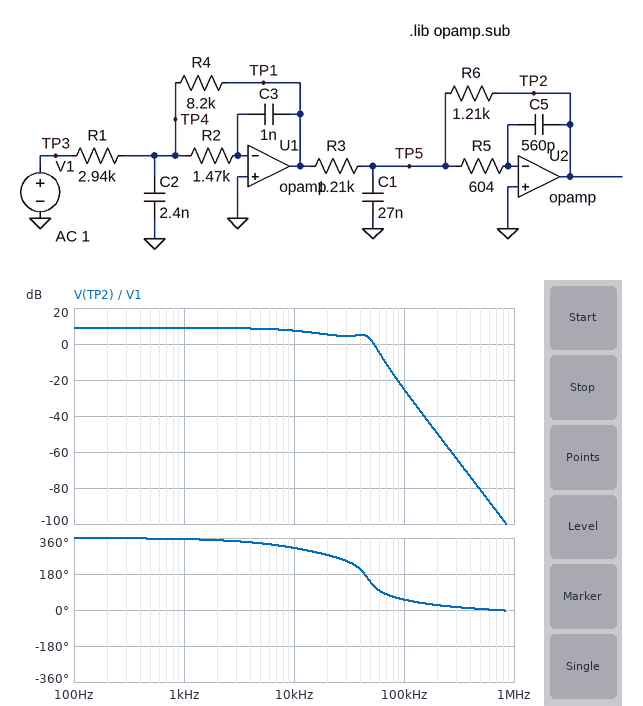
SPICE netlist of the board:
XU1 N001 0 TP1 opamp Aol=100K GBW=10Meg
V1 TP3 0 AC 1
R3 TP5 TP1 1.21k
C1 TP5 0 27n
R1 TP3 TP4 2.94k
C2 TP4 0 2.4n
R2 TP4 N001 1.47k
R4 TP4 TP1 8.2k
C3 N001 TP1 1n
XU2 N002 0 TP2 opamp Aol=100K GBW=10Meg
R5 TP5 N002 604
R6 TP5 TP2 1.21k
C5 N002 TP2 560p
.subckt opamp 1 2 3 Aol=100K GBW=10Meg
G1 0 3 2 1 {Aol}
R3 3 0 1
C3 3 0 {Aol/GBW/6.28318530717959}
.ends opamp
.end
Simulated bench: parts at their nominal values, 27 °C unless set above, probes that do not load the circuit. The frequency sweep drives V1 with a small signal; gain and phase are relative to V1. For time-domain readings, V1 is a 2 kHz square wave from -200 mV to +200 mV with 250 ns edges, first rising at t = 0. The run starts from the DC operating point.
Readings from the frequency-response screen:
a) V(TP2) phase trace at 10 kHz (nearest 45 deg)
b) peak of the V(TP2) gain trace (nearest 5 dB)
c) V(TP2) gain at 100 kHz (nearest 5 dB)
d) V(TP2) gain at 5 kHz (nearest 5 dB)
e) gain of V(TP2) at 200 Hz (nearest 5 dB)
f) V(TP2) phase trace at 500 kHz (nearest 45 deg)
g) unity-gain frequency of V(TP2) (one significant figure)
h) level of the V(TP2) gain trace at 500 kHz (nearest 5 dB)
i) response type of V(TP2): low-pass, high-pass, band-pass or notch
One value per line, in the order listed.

315 deg
10 dB
-25 dB
10 dB
10 dB
0 deg
50 kHz
-80 dB
low-pass
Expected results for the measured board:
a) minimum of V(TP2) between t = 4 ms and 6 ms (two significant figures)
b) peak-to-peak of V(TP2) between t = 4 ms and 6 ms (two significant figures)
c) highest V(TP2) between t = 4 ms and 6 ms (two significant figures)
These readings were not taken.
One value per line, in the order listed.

-560 mV
1.1 V
560 mV
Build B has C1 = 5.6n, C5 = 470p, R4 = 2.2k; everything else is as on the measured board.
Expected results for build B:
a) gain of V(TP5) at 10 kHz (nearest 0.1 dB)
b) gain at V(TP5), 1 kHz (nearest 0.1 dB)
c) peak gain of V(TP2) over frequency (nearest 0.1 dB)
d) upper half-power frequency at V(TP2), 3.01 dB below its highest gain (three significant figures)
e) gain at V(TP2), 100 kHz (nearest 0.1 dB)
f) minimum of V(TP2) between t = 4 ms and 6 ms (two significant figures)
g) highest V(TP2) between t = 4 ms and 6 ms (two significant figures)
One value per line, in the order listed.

-37.1 dB
-57.0 dB
-2.5 dB
54.9 kHz
-11.3 dB
-150 mV
150 mV
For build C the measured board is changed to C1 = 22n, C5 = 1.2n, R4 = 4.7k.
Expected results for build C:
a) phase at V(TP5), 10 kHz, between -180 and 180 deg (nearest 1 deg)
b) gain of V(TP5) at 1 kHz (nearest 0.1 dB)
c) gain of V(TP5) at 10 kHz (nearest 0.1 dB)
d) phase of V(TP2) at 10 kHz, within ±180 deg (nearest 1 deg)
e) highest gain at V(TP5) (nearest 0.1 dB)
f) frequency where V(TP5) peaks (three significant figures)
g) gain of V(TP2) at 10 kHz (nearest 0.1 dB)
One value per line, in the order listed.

-131 deg
-42.6 dB
-22.7 dB
-41 deg
-13.2 dB
32.5 kHz
4.0 dB
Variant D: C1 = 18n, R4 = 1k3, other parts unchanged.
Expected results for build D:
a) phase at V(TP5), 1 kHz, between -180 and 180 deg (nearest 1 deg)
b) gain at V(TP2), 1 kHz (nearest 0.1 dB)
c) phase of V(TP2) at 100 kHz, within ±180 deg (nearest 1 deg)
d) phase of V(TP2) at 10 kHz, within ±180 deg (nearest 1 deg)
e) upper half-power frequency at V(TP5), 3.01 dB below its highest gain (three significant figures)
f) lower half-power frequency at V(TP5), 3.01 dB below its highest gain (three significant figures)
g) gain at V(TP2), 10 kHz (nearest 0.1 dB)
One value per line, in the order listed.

-92 deg
-7.1 dB
91 deg
-18 deg
68.3 kHz
42.3 kHz
-6.9 dB
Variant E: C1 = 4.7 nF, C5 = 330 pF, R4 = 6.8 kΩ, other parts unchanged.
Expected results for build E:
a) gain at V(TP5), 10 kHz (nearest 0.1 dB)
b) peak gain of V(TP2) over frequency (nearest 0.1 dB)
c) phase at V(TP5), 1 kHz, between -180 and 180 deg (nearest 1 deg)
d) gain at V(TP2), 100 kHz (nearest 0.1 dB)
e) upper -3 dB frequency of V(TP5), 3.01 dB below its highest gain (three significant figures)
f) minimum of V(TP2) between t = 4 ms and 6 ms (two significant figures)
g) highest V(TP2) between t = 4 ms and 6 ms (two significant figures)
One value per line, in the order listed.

-31.4 dB
7.3 dB
-95 deg
-11.0 dB
135 kHz
-460 mV
460 mV
